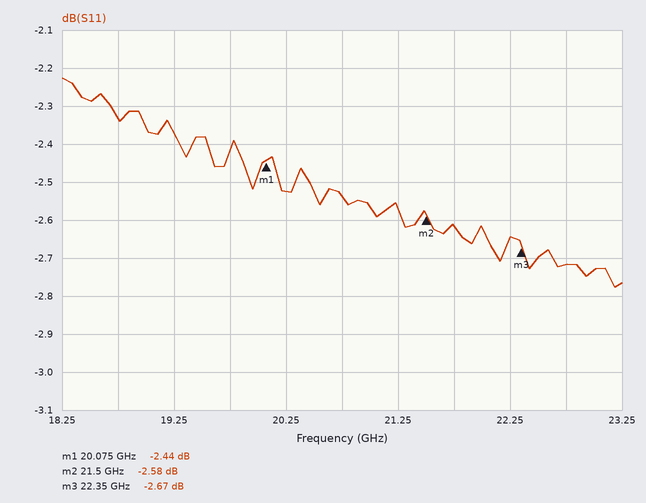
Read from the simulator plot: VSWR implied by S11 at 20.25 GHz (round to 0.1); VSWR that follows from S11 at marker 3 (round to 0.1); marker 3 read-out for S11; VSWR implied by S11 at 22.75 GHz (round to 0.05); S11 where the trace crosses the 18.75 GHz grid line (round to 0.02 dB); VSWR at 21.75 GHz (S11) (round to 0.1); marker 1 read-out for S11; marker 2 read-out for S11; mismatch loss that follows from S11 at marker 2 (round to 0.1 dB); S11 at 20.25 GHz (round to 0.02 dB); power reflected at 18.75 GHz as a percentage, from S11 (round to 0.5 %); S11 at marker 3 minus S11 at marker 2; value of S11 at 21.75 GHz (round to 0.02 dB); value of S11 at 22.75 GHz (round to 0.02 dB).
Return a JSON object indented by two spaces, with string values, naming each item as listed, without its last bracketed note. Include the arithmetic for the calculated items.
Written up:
{
  "VSWR implied by S11 at 20.25 GHz": "|Γ| = 10^(-2.52/20) = 0.7482; VSWR = (1 + 0.7482)/(1 − 0.7482) ≈ 6.9",
  "VSWR that follows from S11 at marker 3": "(1 + 0.7354)/(1 − 0.7354) ≈ 6.6",
  "marker 3 read-out for S11": "-2.67 dB",
  "VSWR implied by S11 at 22.75 GHz": "|Γ| = 10^(-2.72/20) = 0.7311; VSWR = (1 + 0.7311)/(1 − 0.7311) ≈ 6.44, so 6.45 to the nearest 0.05",
  "S11 where the trace crosses the 18.75 GHz grid line": "-2.34 dB",
  "VSWR at 21.75 GHz (S11)": "|Γ| = 10^(-2.62/20) = 0.7396; VSWR = (1 + 0.7396)/(1 − 0.7396) ≈ 6.7",
  "marker 1 read-out for S11": "-2.44 dB",
  "marker 2 read-out for S11": "-2.58 dB",
  "mismatch loss that follows from S11 at marker 2": "−10 log10(1 − 10^(-2.58/10)) ≈ 3.5 dB",
  "S11 at 20.25 GHz": "-2.52 dB",
  "power reflected at 18.75 GHz as a percentage, from S11": "10^(-2.34/10) ≈ 58.3 %, so 58.5 % to the nearest 0.5 %",
  "S11 at marker 3 minus S11 at marker 2": "-2.67 − (-2.58) = -0.09 dB",
  "value of S11 at 21.75 GHz": "-2.62 dB",
  "value of S11 at 22.75 GHz": "-2.72 dB"
}
